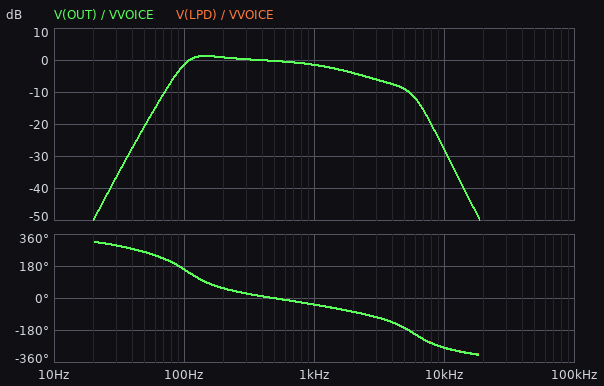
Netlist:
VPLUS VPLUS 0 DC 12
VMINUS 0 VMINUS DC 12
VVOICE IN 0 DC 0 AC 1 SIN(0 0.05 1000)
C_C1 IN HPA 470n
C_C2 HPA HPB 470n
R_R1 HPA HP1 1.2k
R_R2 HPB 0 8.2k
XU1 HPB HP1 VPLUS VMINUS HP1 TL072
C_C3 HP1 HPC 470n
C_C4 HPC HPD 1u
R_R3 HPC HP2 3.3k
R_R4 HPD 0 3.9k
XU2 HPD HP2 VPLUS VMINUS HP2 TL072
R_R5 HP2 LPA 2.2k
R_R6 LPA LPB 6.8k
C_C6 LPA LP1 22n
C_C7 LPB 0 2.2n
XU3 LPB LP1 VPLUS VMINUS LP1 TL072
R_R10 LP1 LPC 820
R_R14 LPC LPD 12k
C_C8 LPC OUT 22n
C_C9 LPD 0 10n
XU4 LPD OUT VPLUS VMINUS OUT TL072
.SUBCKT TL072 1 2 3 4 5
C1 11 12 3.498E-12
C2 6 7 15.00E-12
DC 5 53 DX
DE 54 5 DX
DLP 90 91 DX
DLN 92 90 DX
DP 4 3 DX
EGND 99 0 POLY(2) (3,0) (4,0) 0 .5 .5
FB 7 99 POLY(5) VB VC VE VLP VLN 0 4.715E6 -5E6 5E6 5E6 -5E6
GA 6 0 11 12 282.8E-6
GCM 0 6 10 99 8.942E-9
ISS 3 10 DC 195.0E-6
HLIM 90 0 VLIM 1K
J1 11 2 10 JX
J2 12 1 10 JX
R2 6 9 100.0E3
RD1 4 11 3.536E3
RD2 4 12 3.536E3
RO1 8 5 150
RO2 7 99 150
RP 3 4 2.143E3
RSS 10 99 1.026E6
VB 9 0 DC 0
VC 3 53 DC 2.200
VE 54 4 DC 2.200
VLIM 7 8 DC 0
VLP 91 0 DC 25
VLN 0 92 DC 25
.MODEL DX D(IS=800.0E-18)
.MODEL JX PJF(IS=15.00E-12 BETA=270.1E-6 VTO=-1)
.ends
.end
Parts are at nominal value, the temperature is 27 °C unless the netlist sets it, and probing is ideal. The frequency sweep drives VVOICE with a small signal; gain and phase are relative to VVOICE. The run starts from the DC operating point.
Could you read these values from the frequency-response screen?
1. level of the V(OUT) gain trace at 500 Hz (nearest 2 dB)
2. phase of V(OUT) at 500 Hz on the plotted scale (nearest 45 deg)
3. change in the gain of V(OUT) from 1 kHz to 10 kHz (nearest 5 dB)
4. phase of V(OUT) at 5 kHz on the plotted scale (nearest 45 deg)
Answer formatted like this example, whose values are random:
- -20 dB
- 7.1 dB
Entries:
- 0 dB
- 0 deg
- -25 dB
- -180 deg
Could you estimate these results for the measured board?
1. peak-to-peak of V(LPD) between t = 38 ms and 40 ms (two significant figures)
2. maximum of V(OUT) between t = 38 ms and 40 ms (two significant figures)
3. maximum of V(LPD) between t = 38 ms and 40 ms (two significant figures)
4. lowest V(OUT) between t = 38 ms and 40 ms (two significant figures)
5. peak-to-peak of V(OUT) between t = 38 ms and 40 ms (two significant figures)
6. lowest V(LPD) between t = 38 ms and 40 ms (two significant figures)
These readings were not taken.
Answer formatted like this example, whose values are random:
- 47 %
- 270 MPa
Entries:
- 84 mV
- 42 mV
- 42 mV
- -42 mV
- 84 mV
- -42 mV
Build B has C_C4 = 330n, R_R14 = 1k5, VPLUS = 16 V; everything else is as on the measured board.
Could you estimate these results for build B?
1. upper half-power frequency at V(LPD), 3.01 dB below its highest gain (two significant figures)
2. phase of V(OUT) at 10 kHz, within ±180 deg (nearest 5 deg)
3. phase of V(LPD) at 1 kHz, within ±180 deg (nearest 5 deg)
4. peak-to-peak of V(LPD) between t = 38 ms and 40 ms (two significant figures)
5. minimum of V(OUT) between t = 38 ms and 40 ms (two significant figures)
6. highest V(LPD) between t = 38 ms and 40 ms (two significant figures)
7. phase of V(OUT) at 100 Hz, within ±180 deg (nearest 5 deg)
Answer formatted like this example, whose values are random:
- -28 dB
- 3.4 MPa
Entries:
- 6.8 kHz
- 120 deg
- 0 deg
- 100 mV
- -51 mV
- 51 mV
- -165 deg
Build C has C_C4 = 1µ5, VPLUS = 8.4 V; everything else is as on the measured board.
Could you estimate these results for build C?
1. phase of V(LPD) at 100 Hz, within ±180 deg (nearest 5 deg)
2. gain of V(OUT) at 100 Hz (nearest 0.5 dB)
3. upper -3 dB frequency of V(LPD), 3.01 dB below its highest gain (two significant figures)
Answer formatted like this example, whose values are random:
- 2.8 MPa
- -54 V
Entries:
- 155 deg
- -1.0 dB
- 1.0 kHz
